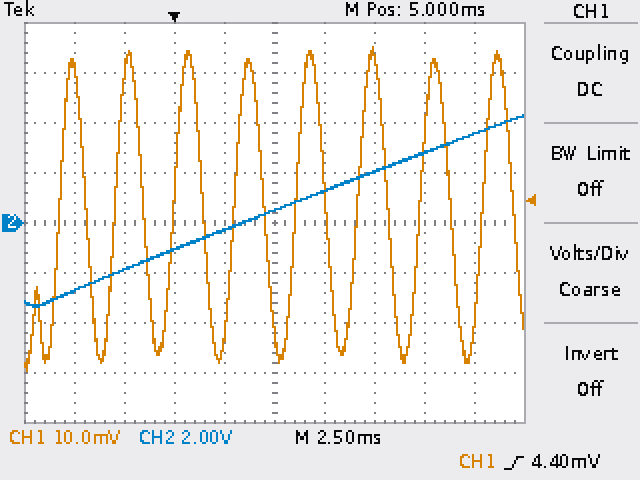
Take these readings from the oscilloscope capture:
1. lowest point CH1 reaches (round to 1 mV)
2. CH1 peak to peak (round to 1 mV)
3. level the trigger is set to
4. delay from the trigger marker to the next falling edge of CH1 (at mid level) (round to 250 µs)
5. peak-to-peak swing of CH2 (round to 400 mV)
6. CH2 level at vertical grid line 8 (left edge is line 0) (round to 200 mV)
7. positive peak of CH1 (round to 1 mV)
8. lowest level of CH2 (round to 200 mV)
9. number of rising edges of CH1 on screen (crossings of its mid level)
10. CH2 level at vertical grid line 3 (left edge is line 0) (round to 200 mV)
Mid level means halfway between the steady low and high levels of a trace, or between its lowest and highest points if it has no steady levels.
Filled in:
-30 mV
65 mV
4.40 mV
1.50 ms
7.6 V
2.8 V
35 mV
-3.4 V
8
-1.0 V
